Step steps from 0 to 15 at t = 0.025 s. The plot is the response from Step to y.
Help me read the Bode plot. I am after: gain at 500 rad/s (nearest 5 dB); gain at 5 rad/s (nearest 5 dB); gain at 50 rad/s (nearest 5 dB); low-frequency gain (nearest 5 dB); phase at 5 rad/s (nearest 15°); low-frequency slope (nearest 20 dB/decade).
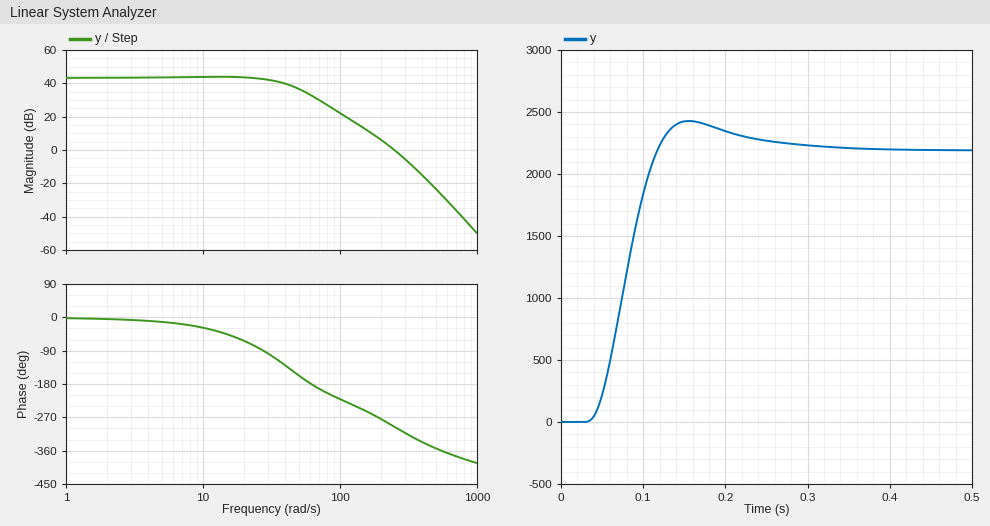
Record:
-25 dB
45 dB
35 dB
45 dB
-15°
0 dB/decade
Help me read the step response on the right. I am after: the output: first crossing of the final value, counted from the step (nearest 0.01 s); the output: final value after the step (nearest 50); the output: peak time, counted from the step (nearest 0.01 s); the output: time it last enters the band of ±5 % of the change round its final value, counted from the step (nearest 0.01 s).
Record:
0.09 s
2200
0.13 s
0.20 s
